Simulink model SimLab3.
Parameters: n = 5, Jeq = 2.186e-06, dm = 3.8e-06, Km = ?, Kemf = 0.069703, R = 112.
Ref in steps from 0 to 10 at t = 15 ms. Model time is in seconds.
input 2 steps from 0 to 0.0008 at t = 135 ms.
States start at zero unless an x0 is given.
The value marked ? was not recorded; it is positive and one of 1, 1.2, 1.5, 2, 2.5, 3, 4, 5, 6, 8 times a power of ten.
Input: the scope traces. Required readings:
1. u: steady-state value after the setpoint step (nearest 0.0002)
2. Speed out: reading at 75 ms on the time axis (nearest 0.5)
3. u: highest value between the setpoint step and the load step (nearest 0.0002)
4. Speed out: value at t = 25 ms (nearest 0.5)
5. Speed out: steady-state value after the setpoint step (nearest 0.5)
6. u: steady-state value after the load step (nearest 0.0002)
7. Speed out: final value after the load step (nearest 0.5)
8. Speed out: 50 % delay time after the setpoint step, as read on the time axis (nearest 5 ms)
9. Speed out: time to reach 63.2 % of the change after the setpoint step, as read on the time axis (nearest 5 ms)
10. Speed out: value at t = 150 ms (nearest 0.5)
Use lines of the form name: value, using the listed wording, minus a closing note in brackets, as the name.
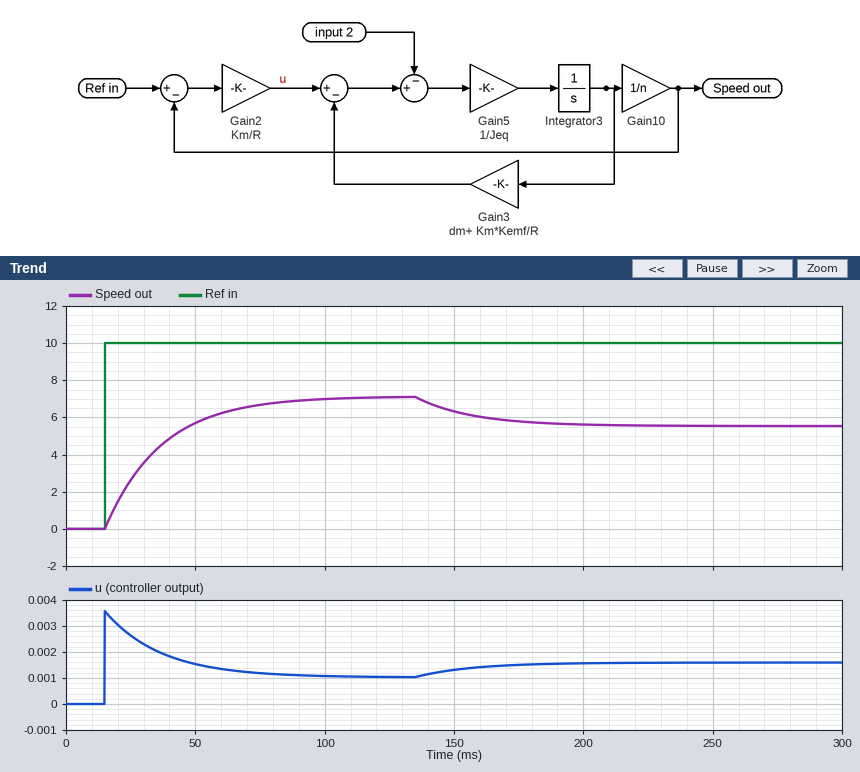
u: steady-state value after the setpoint step: 0.0010
Speed out: reading at 75 ms on the time axis: 6.5
u: highest value between the setpoint step and the load step: 0.0036
Speed out: value at t = 25 ms: 2.5
Speed out: steady-state value after the setpoint step: 7.0
u: steady-state value after the load step: 0.0016
Speed out: final value after the load step: 5.5
Speed out: 50 % delay time after the setpoint step, as read on the time axis: 30 ms
Speed out: time to reach 63.2 % of the change after the setpoint step, as read on the time axis: 35 ms
Speed out: value at t = 150 ms: 6.5
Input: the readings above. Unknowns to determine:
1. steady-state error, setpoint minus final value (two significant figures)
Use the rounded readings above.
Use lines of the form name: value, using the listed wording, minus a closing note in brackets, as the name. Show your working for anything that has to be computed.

steady-state error, setpoint minus final value: 10 - 7 = 3.0
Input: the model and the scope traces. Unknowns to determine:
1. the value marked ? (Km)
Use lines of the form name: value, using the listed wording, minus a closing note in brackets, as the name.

the value marked ?: 0.04
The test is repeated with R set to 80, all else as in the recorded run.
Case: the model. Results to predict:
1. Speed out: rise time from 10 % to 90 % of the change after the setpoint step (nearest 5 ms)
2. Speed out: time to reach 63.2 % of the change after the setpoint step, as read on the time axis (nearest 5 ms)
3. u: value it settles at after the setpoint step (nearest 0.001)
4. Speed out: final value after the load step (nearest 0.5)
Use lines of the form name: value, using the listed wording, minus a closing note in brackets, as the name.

Speed out: rise time from 10 % to 90 % of the change after the setpoint step: 35 ms
Speed out: time to reach 63.2 % of the change after the setpoint step, as read on the time axis: 30 ms
u: value it settles at after the setpoint step: 0.001
Speed out: final value after the load step: 6.0
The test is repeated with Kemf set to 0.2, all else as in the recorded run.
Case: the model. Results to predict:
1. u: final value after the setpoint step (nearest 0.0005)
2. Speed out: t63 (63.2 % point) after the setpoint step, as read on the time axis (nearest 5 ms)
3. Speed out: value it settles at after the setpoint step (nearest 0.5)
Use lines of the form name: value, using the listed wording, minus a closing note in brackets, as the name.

u: final value after the setpoint step: 0.0020
Speed out: t63 (63.2 % point) after the setpoint step, as read on the time axis: 30 ms
Speed out: value it settles at after the setpoint step: 5.0
